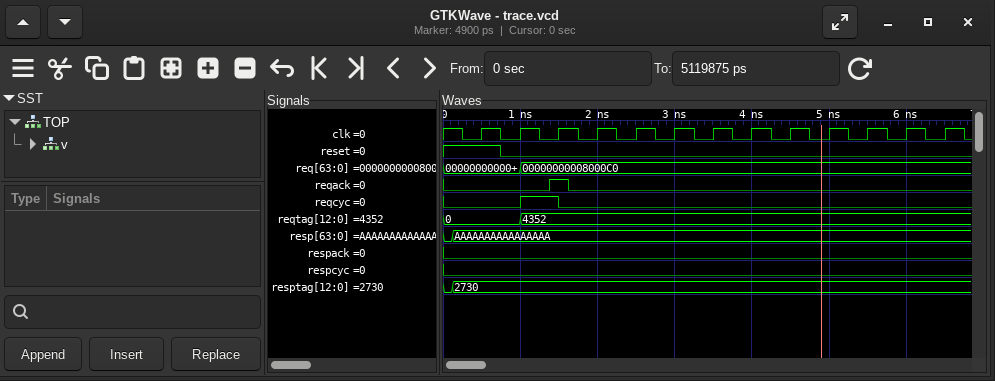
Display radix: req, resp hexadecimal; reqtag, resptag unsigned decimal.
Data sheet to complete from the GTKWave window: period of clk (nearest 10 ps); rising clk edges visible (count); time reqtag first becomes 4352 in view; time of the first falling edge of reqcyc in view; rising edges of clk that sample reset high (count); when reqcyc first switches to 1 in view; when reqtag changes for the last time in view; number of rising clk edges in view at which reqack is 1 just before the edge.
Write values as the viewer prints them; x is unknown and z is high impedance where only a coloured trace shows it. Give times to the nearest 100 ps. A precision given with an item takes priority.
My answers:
500 ps
13
1000 ps
1500 ps
1
1000 ps
1000 ps
1
